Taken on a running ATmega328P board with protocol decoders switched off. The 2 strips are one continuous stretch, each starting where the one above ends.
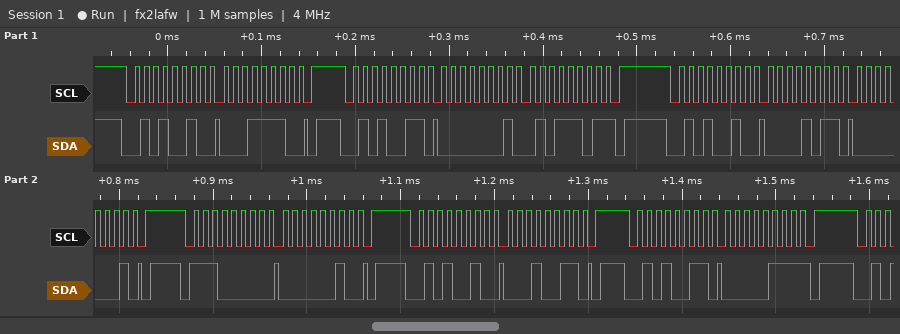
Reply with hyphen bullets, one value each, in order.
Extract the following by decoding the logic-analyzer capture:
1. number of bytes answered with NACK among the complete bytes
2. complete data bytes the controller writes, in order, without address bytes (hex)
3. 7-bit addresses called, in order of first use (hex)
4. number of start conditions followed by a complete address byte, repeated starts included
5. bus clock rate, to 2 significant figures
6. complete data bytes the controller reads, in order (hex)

- 2
- 1E 0B 01 02 13
- 0x29 0x70
- 6
- 100 kHz
- 01 5D 07
